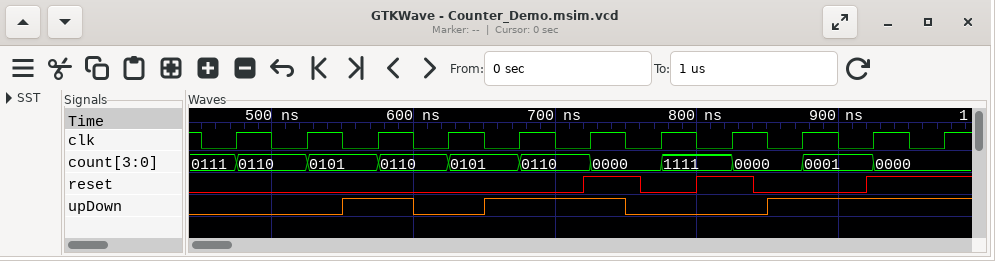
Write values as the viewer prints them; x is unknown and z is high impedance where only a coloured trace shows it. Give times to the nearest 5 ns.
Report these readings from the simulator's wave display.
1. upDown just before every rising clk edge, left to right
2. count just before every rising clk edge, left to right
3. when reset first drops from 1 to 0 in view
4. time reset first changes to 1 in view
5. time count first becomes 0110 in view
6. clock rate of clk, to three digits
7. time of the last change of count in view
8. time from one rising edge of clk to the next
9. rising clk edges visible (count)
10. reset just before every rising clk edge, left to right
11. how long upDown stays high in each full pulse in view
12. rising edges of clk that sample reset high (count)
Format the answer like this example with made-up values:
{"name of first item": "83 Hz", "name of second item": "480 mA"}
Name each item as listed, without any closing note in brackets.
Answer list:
{"upDown just before every rising clk edge, left to right": "0 0 1 0 1 1 0 0 1 1 1", "count just before every rising clk edge, left to right": "0111, 0110, 0101, 0110, 0101, 0110, 0000, 1111, 0000, 0001, 0000", "when reset first drops from 1 to 0 in view": "760 ns", "time reset first changes to 1 in view": "720 ns", "time count first becomes 0110 in view": "475 ns", "clock rate of clk, to three digits": "20.0 MHz", "time of the last change of count in view": "925 ns", "time from one rising edge of clk to the next": "50 ns", "rising clk edges visible": "11", "reset just before every rising clk edge, left to right": "0 0 0 0 0 1 0 1 0 1 1", "how long upDown stays high in each full pulse in view": "50 ns, 100 ns", "rising edges of clk that sample reset high": "4"}
